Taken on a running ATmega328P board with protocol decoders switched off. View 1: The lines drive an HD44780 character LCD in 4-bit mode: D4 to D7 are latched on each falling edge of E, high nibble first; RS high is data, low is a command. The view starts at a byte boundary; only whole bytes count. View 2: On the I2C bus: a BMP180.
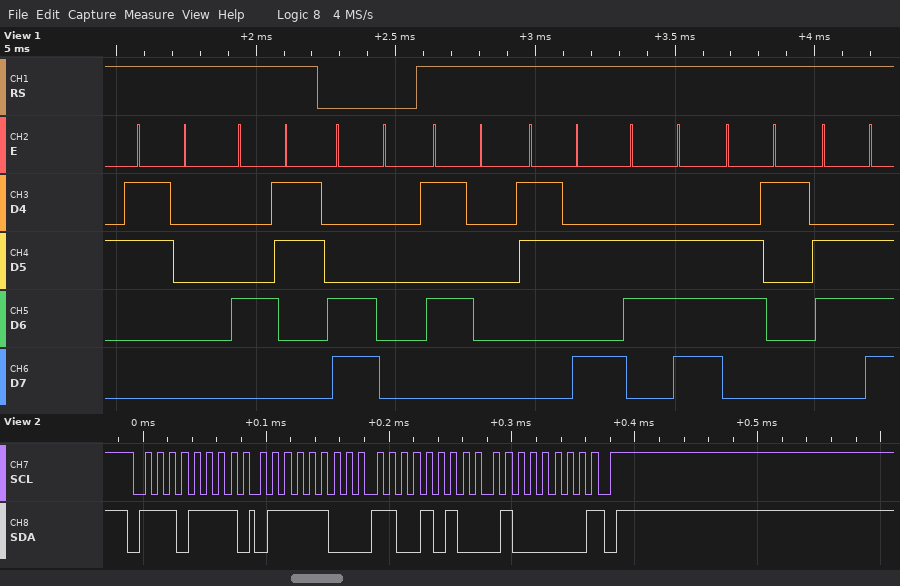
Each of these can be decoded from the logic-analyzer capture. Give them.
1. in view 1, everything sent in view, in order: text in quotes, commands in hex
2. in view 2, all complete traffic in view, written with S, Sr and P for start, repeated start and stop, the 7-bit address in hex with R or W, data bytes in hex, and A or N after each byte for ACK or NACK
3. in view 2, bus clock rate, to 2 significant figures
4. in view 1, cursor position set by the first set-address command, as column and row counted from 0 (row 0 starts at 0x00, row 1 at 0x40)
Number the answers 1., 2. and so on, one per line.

1. "0C" 0xC0 "P:nan"
2. S 77R A 7C A CA A 40 N P
3. 100 kHz
4. column 0, row 1
